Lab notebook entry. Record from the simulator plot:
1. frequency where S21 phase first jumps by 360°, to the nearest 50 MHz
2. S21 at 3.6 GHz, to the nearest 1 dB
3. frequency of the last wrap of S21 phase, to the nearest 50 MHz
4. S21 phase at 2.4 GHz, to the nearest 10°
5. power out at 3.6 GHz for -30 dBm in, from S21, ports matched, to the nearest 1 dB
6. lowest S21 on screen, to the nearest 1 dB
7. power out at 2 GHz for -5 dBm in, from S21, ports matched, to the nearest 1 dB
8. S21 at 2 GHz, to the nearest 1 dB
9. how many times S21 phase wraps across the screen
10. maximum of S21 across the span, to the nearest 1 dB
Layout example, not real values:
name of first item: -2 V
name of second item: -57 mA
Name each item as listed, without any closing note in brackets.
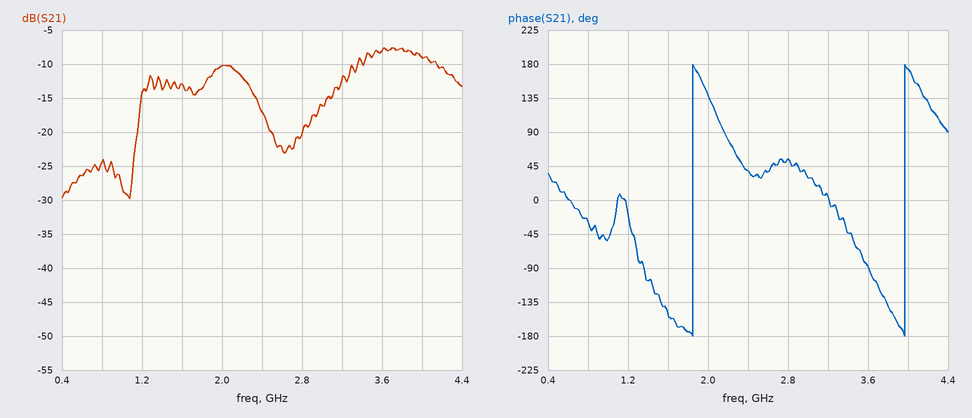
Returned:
frequency where S21 phase first jumps by 360°, to the nearest 50 MHz: 1.85 GHz
S21 at 3.6 GHz, to the nearest 1 dB: -8 dB
frequency of the last wrap of S21 phase, to the nearest 50 MHz: 3.95 GHz
S21 phase at 2.4 GHz, to the nearest 10°: 40°
power out at 3.6 GHz for -30 dBm in, from S21, ports matched, to the nearest 1 dB: -38 dBm
lowest S21 on screen, to the nearest 1 dB: -30 dB
power out at 2 GHz for -5 dBm in, from S21, ports matched, to the nearest 1 dB: -15 dBm
S21 at 2 GHz, to the nearest 1 dB: -10 dB
how many times S21 phase wraps across the screen: 2
maximum of S21 across the span, to the nearest 1 dB: -8 dB
